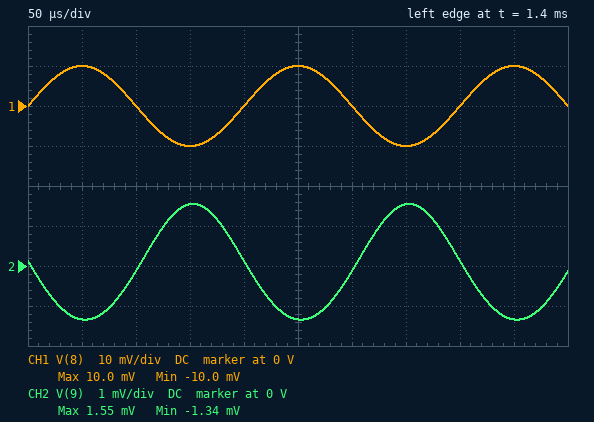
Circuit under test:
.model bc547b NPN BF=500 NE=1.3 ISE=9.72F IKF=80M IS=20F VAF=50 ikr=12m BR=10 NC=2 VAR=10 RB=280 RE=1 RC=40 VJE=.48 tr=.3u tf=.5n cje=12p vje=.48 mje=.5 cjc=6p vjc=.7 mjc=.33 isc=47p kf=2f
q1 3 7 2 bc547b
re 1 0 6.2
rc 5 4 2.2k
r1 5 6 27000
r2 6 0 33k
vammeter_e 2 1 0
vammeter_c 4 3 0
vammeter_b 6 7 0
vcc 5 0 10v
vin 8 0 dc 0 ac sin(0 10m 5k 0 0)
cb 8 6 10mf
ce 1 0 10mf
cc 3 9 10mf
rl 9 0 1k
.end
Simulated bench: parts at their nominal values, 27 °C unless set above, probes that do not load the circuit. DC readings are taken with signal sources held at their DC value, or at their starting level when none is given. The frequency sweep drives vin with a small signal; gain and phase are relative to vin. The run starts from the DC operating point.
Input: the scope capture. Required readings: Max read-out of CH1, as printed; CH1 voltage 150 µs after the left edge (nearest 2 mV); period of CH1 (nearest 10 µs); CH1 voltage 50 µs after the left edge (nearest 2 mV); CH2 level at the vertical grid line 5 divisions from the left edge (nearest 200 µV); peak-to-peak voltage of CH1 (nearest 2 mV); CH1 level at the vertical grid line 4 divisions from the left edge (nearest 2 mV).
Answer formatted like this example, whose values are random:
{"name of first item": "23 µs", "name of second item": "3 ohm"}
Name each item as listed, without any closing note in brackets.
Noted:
{"Max read-out of CH1, as printed": "10.0 mV", "CH1 voltage 150 µs after the left edge": "-10 mV", "period of CH1": "200 µs", "CH1 voltage 50 µs after the left edge": "10 mV", "CH2 level at the vertical grid line 5 divisions from the left edge": "-1.4 mV", "peak-to-peak voltage of CH1": "20 mV", "CH1 level at the vertical grid line 4 divisions from the left edge": "0 V"}
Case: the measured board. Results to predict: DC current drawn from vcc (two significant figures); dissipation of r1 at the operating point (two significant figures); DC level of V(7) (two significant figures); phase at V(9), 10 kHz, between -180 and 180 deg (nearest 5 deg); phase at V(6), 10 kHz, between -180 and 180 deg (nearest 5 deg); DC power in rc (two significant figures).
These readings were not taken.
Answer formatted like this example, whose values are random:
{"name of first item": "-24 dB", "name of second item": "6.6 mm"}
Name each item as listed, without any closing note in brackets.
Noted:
{"DC current drawn from vcc": "4.8 mA", "dissipation of r1 at the operating point": "3.1 mW", "DC level of V(7)": "820 mV", "phase at V(9), 10 kHz, between -180 and 180 deg": "170 deg", "phase at V(6), 10 kHz, between -180 and 180 deg": "0 deg", "DC power in rc": "43 mW"}
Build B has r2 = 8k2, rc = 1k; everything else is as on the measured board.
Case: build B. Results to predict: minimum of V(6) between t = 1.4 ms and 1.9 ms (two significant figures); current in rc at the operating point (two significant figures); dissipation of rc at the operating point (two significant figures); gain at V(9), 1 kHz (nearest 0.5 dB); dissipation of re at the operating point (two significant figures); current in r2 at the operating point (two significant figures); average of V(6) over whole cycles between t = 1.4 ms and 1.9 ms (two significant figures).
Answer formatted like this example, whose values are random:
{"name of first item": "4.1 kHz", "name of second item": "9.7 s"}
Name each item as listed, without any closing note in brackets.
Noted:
{"minimum of V(6) between t = 1.4 ms and 1.9 ms": "830 mV", "current in rc at the operating point": "9.5 mA", "dissipation of rc at the operating point": "90 mW", "gain at V(9), 1 kHz": "-10.5 dB", "dissipation of re at the operating point": "590 µW", "current in r2 at the operating point": "100 µA", "average of V(6) over whole cycles between t = 1.4 ms and 1.9 ms": "840 mV"}
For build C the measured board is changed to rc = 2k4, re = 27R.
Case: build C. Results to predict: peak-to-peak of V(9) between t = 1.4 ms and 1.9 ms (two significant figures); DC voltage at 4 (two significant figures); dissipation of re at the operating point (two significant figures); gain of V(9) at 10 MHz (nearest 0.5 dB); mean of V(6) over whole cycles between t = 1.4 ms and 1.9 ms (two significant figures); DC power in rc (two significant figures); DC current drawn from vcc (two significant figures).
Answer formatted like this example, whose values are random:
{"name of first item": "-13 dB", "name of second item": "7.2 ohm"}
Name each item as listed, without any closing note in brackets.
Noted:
{"peak-to-peak of V(9) between t = 1.4 ms and 1.9 ms": "2.8 mV", "DC voltage at 4": "310 mV", "dissipation of re at the operating point": "510 µW", "gain of V(9) at 10 MHz": "-35.0 dB", "mean of V(6) over whole cycles between t = 1.4 ms and 1.9 ms": "900 mV", "DC power in rc": "39 mW", "DC current drawn from vcc": "4.4 mA"}
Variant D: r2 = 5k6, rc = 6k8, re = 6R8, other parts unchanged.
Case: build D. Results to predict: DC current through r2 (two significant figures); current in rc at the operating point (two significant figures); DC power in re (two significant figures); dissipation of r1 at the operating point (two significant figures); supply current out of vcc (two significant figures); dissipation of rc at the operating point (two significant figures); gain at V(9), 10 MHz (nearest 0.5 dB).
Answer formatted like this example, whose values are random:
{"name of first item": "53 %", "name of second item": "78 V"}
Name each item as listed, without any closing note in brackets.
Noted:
{"DC current through r2": "130 µA", "current in rc at the operating point": "1.5 mA", "DC power in re": "19 µW", "dissipation of r1 at the operating point": "3.2 mW", "supply current out of vcc": "1.8 mA", "dissipation of rc at the operating point": "14 mW", "gain at V(9), 10 MHz": "-30.0 dB"}
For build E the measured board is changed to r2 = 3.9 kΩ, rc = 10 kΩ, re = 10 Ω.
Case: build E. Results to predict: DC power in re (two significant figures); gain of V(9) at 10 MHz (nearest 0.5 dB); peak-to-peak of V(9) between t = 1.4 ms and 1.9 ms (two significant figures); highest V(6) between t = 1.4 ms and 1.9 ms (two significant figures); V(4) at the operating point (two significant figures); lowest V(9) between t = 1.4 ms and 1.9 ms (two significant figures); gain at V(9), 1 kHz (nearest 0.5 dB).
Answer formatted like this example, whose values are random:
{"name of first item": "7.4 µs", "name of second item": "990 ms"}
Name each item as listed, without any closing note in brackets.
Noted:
{"DC power in re": "13 µW", "gain of V(9) at 10 MHz": "-28.0 dB", "peak-to-peak of V(9) between t = 1.4 ms and 1.9 ms": "3.3 mV", "highest V(6) between t = 1.4 ms and 1.9 ms": "730 mV", "V(4) at the operating point": "71 mV", "lowest V(9) between t = 1.4 ms and 1.9 ms": "-1.5 mV", "gain at V(9), 1 kHz": "-15.5 dB"}
